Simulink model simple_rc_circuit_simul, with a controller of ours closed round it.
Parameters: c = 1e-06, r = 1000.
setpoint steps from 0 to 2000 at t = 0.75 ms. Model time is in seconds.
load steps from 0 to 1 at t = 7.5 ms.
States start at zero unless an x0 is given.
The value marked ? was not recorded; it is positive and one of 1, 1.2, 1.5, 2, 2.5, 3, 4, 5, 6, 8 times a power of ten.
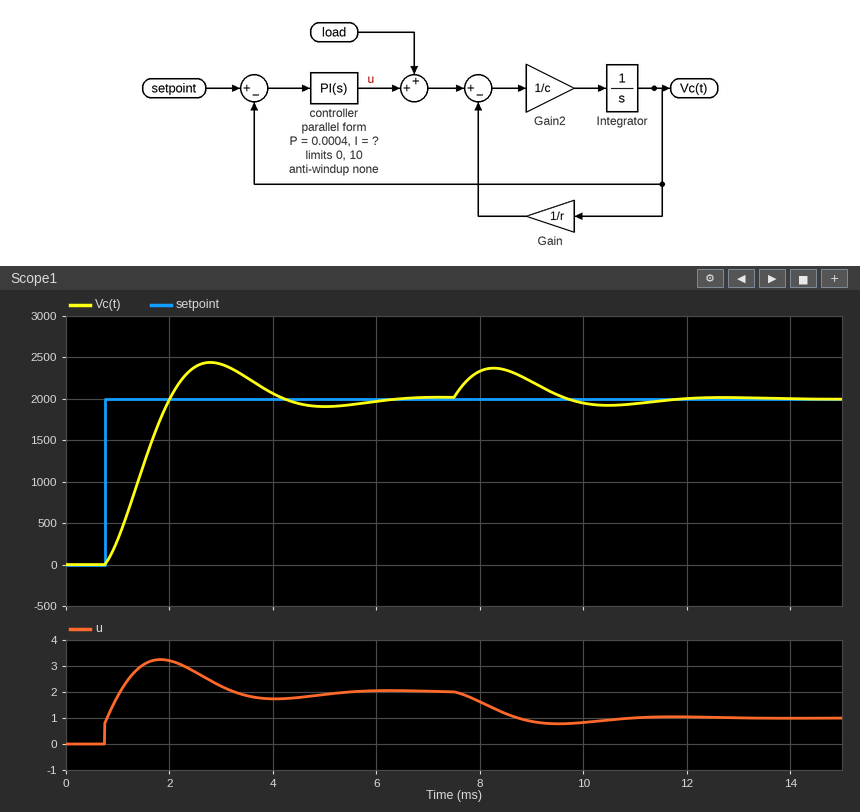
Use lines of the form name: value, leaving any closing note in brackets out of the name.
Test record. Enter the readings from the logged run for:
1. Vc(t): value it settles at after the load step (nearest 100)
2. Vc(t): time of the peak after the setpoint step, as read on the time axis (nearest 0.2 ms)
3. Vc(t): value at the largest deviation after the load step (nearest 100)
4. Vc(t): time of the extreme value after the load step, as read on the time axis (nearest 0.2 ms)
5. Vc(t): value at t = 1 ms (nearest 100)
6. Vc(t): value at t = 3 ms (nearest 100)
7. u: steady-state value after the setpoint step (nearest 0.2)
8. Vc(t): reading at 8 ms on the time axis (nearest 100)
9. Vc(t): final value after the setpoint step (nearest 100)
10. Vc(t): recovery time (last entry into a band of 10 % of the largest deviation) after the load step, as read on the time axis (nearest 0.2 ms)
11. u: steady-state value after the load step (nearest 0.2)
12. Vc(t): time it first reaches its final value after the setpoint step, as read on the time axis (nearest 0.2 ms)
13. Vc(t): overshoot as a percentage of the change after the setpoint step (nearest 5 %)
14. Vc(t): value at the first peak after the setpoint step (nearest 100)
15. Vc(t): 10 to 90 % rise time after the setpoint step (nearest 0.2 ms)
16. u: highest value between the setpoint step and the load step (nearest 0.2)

Vc(t): value it settles at after the load step: 2000
Vc(t): time of the peak after the setpoint step, as read on the time axis: 2.8 ms
Vc(t): value at the largest deviation after the load step: 2400
Vc(t): time of the extreme value after the load step, as read on the time axis: 8.2 ms
Vc(t): value at t = 1 ms: 300
Vc(t): value at t = 3 ms: 2400
u: steady-state value after the setpoint step: 2.0
Vc(t): reading at 8 ms on the time axis: 2300
Vc(t): final value after the setpoint step: 2000
Vc(t): recovery time (last entry into a band of 10 % of the largest deviation) after the load step, as read on the time axis: 11.4 ms
u: steady-state value after the load step: 1.0
Vc(t): time it first reaches its final value after the setpoint step, as read on the time axis: 2.0 ms
Vc(t): overshoot as a percentage of the change after the setpoint step: 20 %
Vc(t): value at the first peak after the setpoint step: 2400
Vc(t): 10 to 90 % rise time after the setpoint step: 1.0 ms
u: highest value between the setpoint step and the load step: 3.2
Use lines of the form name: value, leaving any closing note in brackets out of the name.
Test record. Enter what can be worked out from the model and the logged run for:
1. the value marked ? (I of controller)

the value marked ?: 2.5
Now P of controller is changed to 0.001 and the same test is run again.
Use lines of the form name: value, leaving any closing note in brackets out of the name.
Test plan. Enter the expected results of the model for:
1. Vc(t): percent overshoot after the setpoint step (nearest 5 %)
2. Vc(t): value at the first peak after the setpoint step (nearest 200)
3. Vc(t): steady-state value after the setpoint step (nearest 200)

Vc(t): percent overshoot after the setpoint step: 10 %
Vc(t): value at the first peak after the setpoint step: 2200
Vc(t): steady-state value after the setpoint step: 2000
